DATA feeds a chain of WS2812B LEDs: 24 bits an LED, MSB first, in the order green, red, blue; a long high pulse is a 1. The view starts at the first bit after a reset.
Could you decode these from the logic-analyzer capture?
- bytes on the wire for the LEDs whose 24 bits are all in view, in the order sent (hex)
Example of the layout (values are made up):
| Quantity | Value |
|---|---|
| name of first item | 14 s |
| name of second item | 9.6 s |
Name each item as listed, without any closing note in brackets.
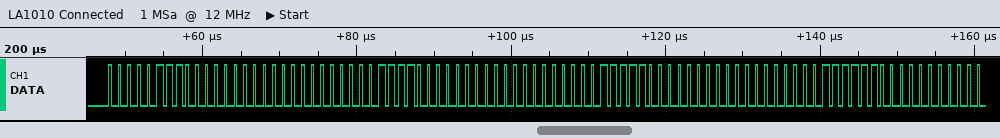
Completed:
| Quantity | Value |
|---|---|
| bytes on the wire for the LEDs whose 24 bits are all in view, in the order sent | 07 00 00 0F 00 00 1F 00 00 |
